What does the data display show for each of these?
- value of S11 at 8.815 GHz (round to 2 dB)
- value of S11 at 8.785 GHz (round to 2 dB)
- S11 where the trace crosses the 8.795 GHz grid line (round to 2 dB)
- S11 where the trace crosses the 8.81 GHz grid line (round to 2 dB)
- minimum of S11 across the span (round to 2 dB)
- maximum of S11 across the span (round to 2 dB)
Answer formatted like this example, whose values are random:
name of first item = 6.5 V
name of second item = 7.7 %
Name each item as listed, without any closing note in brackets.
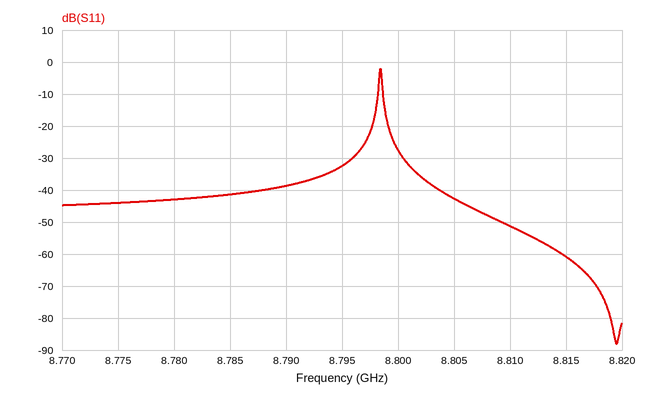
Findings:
value of S11 at 8.815 GHz = -60 dB
value of S11 at 8.785 GHz = -42 dB
S11 where the trace crosses the 8.795 GHz grid line = -32 dB
S11 where the trace crosses the 8.81 GHz grid line = -52 dB
minimum of S11 across the span = -88 dB
maximum of S11 across the span = -2 dB
